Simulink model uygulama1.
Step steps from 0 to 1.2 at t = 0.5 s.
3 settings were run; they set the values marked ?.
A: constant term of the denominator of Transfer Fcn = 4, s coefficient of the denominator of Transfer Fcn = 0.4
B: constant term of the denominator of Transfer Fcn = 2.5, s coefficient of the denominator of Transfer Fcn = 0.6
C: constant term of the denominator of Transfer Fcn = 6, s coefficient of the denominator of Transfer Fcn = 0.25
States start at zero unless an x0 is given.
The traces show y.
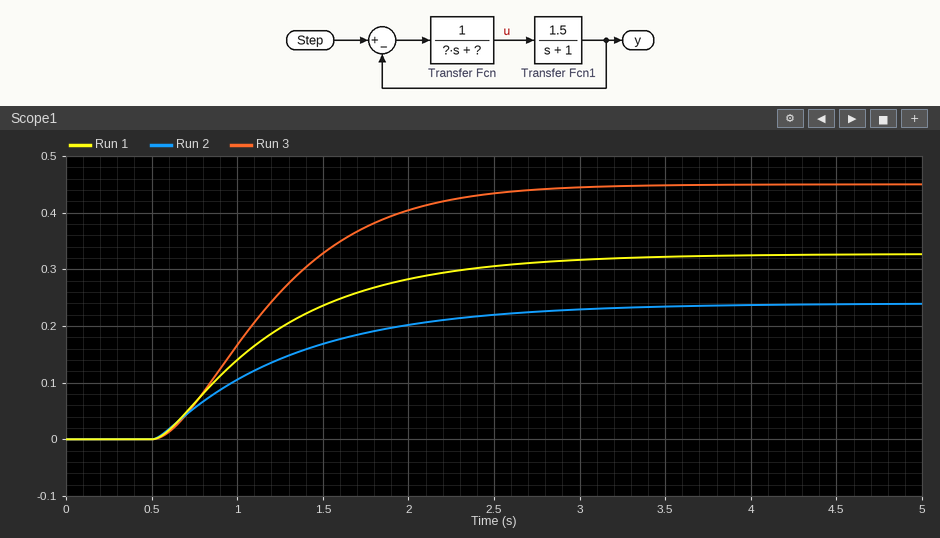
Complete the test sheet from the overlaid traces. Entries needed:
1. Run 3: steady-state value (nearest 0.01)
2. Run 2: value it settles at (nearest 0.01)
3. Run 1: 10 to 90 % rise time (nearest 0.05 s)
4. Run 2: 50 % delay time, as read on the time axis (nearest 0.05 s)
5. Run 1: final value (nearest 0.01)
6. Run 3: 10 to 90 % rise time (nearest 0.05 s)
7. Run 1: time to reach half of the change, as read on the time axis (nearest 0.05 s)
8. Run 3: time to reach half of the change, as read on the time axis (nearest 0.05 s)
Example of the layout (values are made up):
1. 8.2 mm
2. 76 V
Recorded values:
1. 0.45
2. 0.24
3. 1.55 s
4. 1.10 s
5. 0.33
6. 1.30 s
7. 1.10 s
8. 1.15 s
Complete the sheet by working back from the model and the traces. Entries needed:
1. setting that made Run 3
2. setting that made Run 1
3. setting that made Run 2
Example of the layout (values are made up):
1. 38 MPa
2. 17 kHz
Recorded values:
1. B
2. A
3. C
